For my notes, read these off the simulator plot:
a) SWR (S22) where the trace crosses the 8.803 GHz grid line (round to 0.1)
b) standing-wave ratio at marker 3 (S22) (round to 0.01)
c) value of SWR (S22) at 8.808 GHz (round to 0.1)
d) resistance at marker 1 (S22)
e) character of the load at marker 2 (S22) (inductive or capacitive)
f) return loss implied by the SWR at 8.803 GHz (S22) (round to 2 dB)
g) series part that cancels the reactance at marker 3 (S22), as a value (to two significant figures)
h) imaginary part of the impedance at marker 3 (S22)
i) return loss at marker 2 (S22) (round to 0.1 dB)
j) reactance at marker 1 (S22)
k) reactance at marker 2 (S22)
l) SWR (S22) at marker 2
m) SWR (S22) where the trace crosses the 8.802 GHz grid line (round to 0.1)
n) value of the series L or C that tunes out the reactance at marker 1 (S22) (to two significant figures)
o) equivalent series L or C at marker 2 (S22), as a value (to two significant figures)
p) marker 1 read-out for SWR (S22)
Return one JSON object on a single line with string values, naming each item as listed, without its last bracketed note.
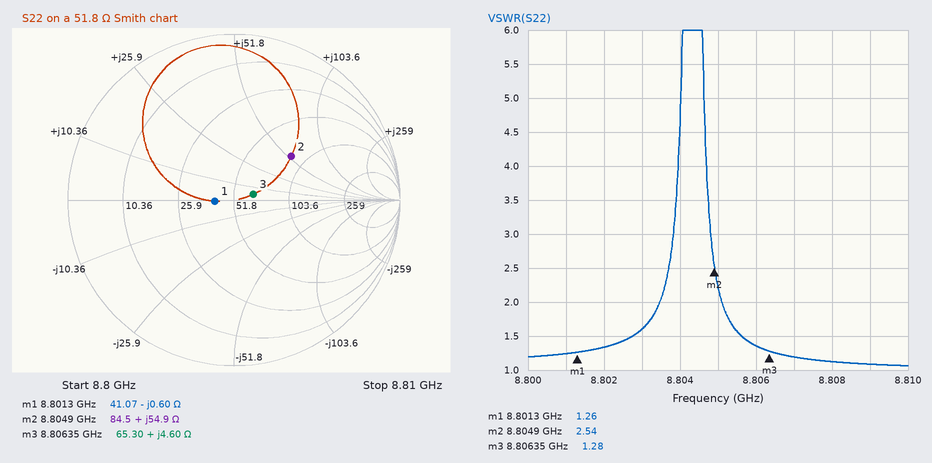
{"SWR (S22) where the trace crosses the 8.803 GHz grid line": "1.6", "standing-wave ratio at marker 3 (S22)": "1.28", "value of SWR (S22) at 8.808 GHz": "1.1", "resistance at marker 1": "41.07 Ω", "character of the load at marker 2 (S22)": "inductive", "return loss implied by the SWR at 8.803 GHz (S22)": "12 dB", "series part that cancels the reactance at marker 3 (S22), as a value": "3.9 pF", "imaginary part of the impedance at marker 3": "+4.60 Ω", "return loss at marker 2 (S22)": "7.2 dB", "reactance at marker 1": "-0.60 Ω", "reactance at marker 2": "+54.9 Ω", "SWR (S22) at marker 2": "2.54", "SWR (S22) where the trace crosses the 8.802 GHz grid line": "1.3", "value of the series L or C that tunes out the reactance at marker 1 (S22)": "11 pH", "equivalent series L or C at marker 2 (S22), as a value": "990 pH", "marker 1 read-out for SWR": "1.26"}
